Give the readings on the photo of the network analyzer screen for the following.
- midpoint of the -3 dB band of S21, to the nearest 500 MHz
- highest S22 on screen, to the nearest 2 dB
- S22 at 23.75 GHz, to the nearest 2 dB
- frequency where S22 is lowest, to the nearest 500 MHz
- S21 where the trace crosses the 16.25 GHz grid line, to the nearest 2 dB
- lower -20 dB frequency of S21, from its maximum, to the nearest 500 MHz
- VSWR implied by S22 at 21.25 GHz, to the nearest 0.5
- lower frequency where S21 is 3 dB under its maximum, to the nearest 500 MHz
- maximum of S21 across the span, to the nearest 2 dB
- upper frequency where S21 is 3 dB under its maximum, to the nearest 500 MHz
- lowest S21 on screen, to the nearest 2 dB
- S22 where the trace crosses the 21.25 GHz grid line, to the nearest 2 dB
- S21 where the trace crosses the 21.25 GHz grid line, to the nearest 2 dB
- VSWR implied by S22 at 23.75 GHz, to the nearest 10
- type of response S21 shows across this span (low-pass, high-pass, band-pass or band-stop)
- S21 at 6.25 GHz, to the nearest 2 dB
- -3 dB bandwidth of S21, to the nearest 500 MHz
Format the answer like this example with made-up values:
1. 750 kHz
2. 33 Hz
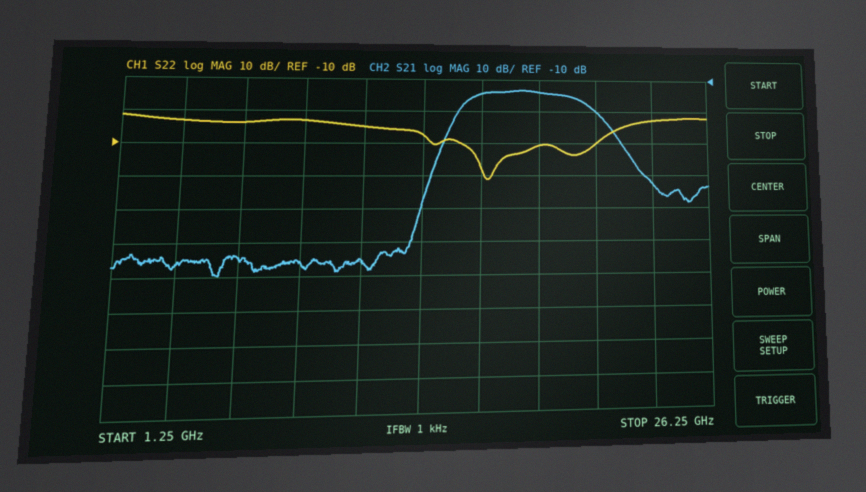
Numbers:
1. 18.0 GHz
2. -2 dB
3. -2 dB
4. 16.5 GHz
5. -14 dB
6. 14.5 GHz
7. 2.0
8. 15.5 GHz
9. -14 dB
10. 20.5 GHz
11. -70 dB
12. -10 dB
13. -20 dB
14. 10
15. band-pass
16. -64 dB
17. 5.0 GHz
